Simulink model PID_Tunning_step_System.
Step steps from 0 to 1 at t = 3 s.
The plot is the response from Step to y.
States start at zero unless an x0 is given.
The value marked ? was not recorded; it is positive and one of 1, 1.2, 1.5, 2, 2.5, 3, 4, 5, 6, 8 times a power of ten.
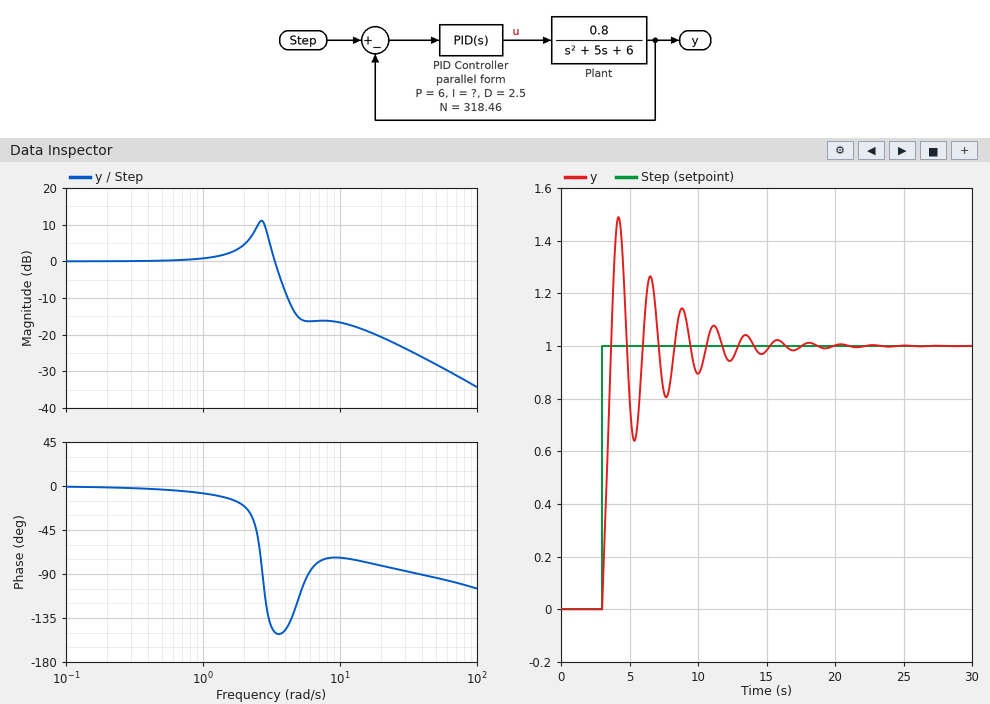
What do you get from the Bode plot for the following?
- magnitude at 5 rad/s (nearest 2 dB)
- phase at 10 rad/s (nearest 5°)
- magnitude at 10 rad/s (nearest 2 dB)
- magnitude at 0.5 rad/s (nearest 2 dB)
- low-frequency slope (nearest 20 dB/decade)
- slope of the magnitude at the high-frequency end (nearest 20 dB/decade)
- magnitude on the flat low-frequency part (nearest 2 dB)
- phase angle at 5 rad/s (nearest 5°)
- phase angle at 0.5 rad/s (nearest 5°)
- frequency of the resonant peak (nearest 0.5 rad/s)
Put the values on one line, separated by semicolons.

-16 dB; -75°; -16 dB; 0 dB; 0 dB/decade; -20 dB/decade; 0 dB; -115°; -5°; 2.5 rad/s
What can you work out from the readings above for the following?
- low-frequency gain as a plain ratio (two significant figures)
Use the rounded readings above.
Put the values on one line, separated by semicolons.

1.0
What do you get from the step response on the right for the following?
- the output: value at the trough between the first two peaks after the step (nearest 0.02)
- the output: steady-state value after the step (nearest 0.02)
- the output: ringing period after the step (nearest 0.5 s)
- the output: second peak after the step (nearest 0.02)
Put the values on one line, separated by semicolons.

0.64; 1.00; 2.5 s; 1.26
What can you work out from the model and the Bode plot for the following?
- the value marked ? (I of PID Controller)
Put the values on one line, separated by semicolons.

60
